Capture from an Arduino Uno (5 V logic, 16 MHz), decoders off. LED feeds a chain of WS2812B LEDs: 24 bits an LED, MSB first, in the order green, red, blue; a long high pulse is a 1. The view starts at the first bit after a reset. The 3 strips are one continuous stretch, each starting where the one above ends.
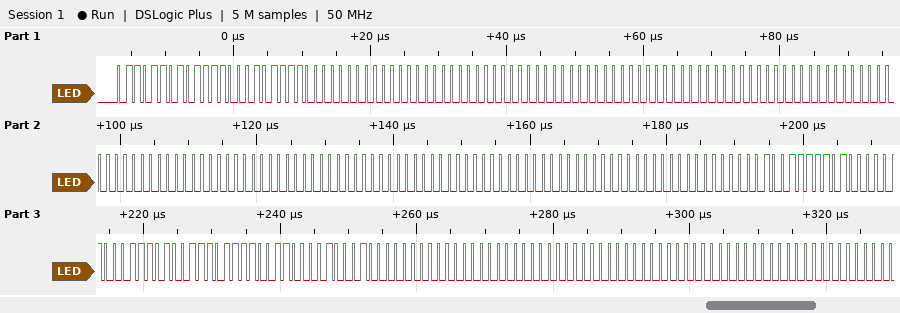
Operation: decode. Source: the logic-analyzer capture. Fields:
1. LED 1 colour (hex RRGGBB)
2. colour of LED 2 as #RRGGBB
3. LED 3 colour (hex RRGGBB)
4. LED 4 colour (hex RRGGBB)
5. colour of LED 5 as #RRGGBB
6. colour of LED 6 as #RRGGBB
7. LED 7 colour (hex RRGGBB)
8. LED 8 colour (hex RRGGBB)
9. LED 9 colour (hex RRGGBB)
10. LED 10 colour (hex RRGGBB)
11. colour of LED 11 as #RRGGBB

#786DBC
#000000
#000000
#000000
#000000
#000000
#000000
#A04F8E
#E69D11
#000000
#000000
